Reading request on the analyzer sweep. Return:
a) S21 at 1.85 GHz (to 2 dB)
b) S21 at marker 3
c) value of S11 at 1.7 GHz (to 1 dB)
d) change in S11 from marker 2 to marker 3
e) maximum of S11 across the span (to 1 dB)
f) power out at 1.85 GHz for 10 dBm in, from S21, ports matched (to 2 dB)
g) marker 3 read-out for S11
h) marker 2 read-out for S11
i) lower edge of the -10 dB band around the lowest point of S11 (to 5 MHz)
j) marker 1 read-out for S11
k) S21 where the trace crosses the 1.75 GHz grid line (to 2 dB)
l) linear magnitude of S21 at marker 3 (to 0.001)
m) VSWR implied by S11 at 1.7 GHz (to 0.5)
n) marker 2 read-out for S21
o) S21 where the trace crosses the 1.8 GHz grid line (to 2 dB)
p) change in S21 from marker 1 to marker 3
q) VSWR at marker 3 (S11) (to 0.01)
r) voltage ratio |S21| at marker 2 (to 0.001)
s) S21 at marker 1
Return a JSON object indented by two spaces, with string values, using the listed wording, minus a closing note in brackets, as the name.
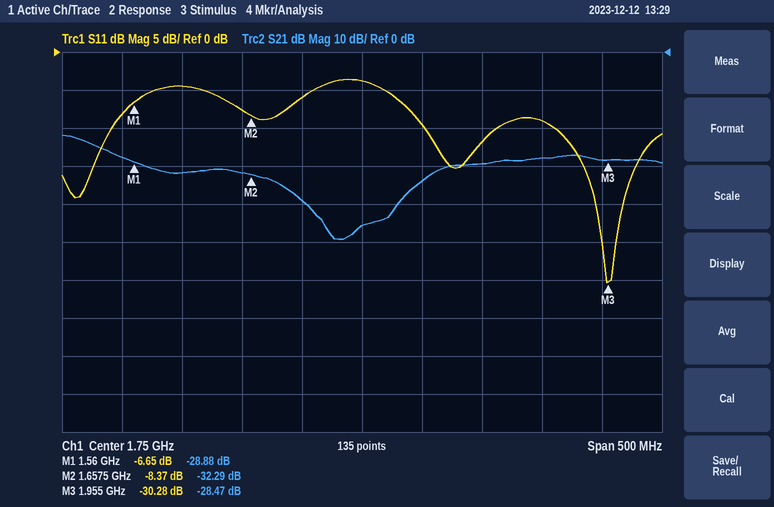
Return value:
{
  "S21 at 1.85 GHz": "-30 dB",
  "S21 at marker 3": "-28.47 dB",
  "value of S11 at 1.7 GHz": "-6 dB",
  "change in S11 from marker 2 to marker 3": "-21.91 dB",
  "maximum of S11 across the span": "-4 dB",
  "power out at 1.85 GHz for 10 dBm in, from S21, ports matched": "-20 dBm",
  "marker 3 read-out for S11": "-30.28 dB",
  "marker 2 read-out for S11": "-8.37 dB",
  "lower edge of the -10 dB band around the lowest point of S11": "1.910 GHz",
  "marker 1 read-out for S11": "-6.65 dB",
  "S21 where the trace crosses the 1.75 GHz grid line": "-46 dB",
  "linear magnitude of S21 at marker 3": "0.038",
  "VSWR implied by S11 at 1.7 GHz": "3.0",
  "marker 2 read-out for S21": "-32.29 dB",
  "S21 where the trace crosses the 1.8 GHz grid line": "-34 dB",
  "change in S21 from marker 1 to marker 3": "0.41 dB",
  "VSWR at marker 3 (S11)": "1.06",
  "voltage ratio |S21| at marker 2": "0.024",
  "S21 at marker 1": "-28.88 dB"
}
